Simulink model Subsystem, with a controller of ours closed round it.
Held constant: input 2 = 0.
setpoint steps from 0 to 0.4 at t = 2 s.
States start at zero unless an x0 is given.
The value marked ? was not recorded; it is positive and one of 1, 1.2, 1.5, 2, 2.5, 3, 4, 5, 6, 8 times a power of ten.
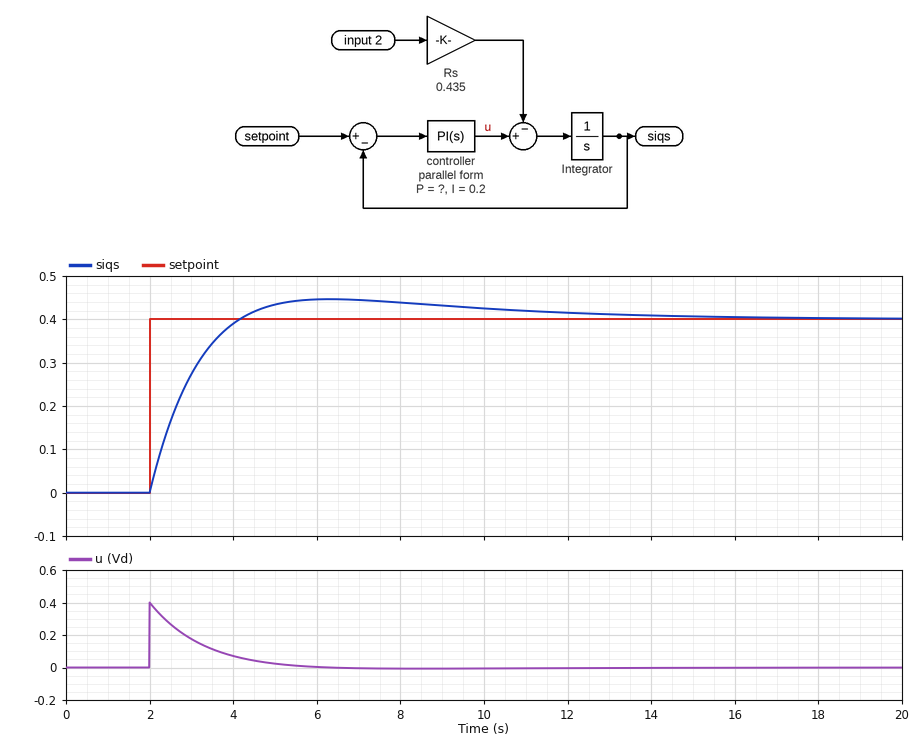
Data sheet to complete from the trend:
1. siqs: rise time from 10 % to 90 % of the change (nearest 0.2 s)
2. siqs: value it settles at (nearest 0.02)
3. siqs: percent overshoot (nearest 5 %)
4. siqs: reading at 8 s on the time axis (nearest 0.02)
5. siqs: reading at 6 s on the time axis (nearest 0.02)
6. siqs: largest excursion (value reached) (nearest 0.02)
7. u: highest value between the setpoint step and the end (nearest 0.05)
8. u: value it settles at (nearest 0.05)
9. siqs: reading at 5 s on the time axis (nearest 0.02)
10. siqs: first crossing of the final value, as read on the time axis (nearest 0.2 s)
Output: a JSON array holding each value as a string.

["1.6 s", "0.40", "10 %", "0.44", "0.44", "0.44", "0.40", "0.00", "0.44", "4.2 s"]
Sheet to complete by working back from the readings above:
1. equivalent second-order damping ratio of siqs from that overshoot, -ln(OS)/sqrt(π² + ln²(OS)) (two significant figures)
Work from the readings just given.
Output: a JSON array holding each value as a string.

["0.59"]
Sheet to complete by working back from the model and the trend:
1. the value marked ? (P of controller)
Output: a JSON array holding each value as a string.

["1"]
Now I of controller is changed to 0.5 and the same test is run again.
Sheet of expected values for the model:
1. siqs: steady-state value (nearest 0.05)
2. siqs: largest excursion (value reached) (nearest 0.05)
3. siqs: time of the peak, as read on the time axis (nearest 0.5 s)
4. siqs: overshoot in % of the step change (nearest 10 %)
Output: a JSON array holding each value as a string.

["0.40", "0.50", "5.0 s", "20 %"]
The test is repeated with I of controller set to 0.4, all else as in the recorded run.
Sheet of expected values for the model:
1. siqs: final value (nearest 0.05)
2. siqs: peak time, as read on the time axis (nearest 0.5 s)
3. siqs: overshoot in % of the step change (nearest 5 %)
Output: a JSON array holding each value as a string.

["0.40", "5.5 s", "20 %"]
